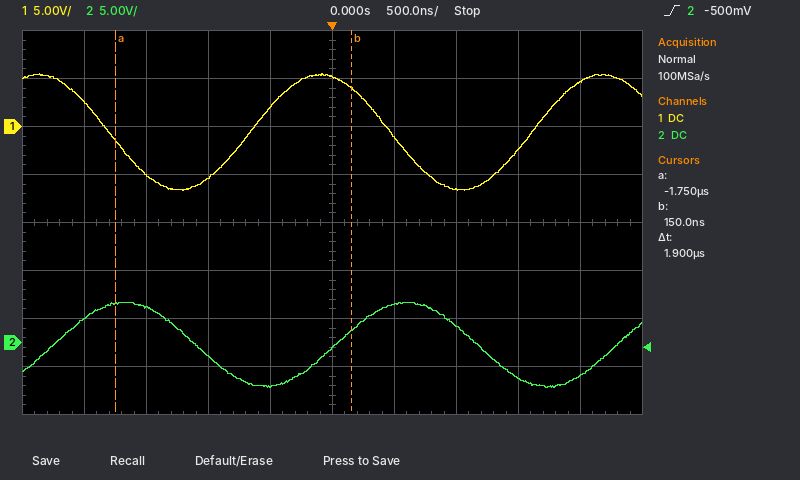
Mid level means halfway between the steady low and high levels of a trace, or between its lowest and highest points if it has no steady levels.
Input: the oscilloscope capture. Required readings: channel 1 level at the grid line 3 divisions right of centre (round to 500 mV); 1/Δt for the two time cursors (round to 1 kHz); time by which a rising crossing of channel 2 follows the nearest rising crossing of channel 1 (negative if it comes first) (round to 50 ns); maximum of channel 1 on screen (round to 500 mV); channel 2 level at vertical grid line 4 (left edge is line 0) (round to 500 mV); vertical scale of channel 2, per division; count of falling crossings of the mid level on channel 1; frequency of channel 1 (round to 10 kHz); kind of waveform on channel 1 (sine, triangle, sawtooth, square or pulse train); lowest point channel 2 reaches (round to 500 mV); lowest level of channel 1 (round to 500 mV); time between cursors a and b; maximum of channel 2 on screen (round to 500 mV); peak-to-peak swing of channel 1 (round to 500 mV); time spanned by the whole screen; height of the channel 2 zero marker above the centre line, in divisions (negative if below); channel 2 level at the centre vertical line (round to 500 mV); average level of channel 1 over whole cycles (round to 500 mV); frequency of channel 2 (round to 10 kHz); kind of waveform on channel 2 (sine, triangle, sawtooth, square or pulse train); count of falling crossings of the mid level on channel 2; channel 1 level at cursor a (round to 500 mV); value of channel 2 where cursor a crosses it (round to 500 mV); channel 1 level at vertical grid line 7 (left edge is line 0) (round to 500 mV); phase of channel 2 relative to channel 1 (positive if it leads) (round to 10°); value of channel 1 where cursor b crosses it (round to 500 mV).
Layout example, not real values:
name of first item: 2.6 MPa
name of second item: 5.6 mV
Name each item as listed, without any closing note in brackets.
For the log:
channel 1 level at the grid line 3 divisions right of centre: -2.5 V
1/Δt for the two time cursors: 526 kHz
time by which a rising crossing of channel 2 follows the nearest rising crossing of channel 1 (negative if it comes first): +700 ns
maximum of channel 1 on screen: 5.5 V
channel 2 level at vertical grid line 4 (left edge is line 0): -4.5 V
vertical scale of channel 2, per division: 5 V
count of falling crossings of the mid level on channel 1: 2
frequency of channel 1: 440 kHz
kind of waveform on channel 1: sine
lowest point channel 2 reaches: -4.5 V
lowest level of channel 1: -6.5 V
time between cursors a and b: 1.9 µs
maximum of channel 2 on screen: 4.0 V
peak-to-peak swing of channel 1: 12.0 V
time spanned by the whole screen: 5 µs
height of the channel 2 zero marker above the centre line, in divisions: -2.5 div
channel 2 level at the centre vertical line: -500 mV
average level of channel 1 over whole cycles: -500 mV
frequency of channel 2: 440 kHz
kind of waveform on channel 2: sine
count of falling crossings of the mid level on channel 2: 2
channel 1 level at cursor a: -1.5 V
value of channel 2 where cursor a crosses it: 4.0 V
channel 1 level at vertical grid line 7 (left edge is line 0): -6.5 V
phase of channel 2 relative to channel 1 (positive if it leads): -110°
value of channel 1 where cursor b crosses it: 4.0 V
